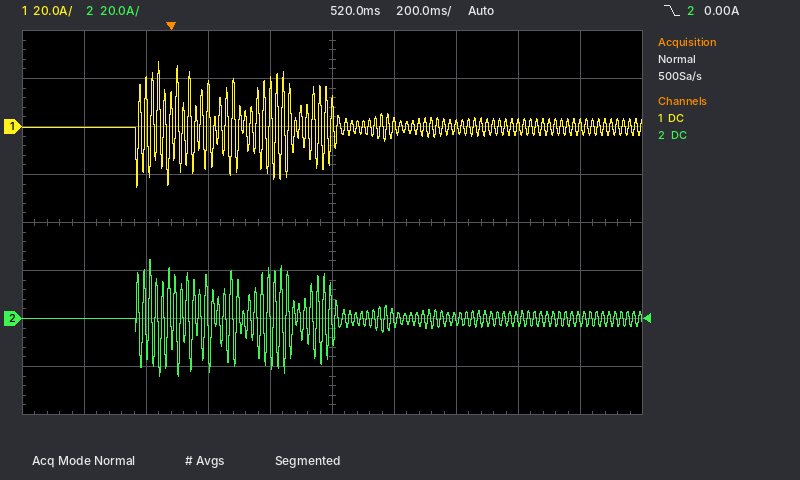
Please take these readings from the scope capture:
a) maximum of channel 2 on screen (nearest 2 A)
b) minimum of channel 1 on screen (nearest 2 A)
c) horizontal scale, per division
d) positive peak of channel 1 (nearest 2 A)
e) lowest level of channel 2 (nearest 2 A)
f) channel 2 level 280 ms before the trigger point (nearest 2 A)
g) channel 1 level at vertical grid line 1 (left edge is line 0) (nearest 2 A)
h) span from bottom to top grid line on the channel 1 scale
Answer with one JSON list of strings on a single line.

["24 A", "-26 A", "200 ms", "28 A", "-24 A", "0 A", "0 A", "160 A"]
